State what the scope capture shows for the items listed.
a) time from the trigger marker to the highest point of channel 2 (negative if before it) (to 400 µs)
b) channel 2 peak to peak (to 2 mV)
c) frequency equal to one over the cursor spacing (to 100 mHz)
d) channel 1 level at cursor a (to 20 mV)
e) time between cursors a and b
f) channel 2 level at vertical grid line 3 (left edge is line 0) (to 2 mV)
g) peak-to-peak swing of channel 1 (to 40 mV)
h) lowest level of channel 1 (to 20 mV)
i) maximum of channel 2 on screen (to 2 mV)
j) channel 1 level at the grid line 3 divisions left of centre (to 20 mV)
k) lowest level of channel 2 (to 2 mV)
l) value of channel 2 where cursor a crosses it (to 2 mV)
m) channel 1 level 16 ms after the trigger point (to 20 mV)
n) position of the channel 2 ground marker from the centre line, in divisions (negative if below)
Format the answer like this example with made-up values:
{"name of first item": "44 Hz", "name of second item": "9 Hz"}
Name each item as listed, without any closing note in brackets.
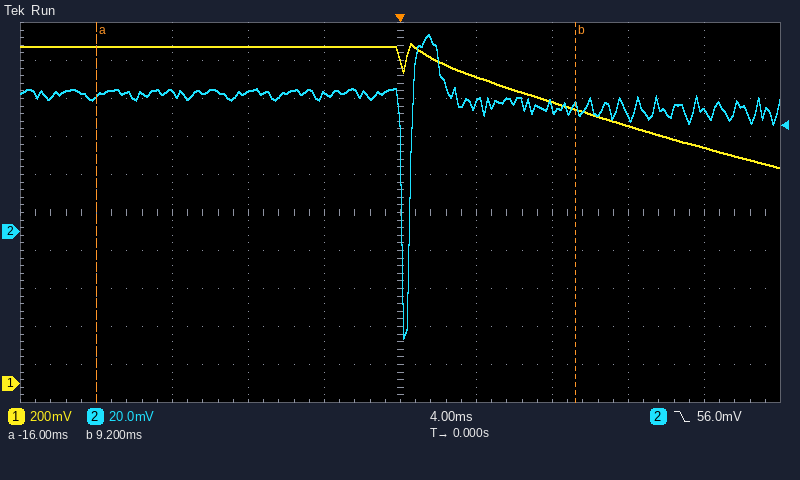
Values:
{"time from the trigger marker to the highest point of channel 2 (negative if before it)": "+1.6 ms", "channel 2 peak to peak": "160 mV", "frequency equal to one over the cursor spacing": "39.7 Hz", "channel 1 level at cursor a": "1.78 V", "time between cursors a and b": "25.2 ms", "channel 2 level at vertical grid line 3 (left edge is line 0)": "74 mV", "peak-to-peak swing of channel 1": "640 mV", "lowest level of channel 1": "1.14 V", "maximum of channel 2 on screen": "104 mV", "channel 1 level at the grid line 3 divisions left of centre": "1.78 V", "lowest level of channel 2": "-56 mV", "value of channel 2 where cursor a crosses it": "72 mV", "channel 1 level 16 ms after the trigger point": "1.24 V", "position of the channel 2 ground marker from the centre line, in divisions": "-0.5 div"}
